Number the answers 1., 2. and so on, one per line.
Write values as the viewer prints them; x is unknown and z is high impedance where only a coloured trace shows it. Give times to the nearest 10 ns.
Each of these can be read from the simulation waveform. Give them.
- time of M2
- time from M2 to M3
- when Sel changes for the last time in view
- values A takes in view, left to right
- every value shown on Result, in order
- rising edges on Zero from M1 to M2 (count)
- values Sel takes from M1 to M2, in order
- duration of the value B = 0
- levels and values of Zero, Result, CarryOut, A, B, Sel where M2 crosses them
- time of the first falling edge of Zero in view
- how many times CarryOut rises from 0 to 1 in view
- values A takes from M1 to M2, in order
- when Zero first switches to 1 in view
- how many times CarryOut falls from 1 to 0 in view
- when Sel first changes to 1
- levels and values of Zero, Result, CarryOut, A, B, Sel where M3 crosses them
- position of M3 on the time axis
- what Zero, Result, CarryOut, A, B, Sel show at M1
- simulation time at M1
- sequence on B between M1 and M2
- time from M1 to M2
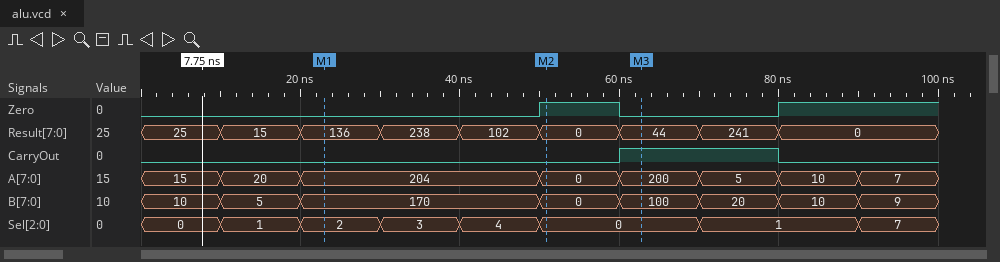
1. 50 ns
2. 10 ns
3. 90 ns
4. 15, 20, 204, 0, 200, 5, 10, 7
5. 25, 15, 136, 238, 102, 0, 44, 241, 0
6. 1
7. 2, 3, 4, 0
8. 10 ns
9. Zero=1, Result=0, CarryOut=0, A=0, B=0, Sel=0
10. 60 ns
11. 1
12. 204, 0
13. 50 ns
14. 1
15. 10 ns
16. Zero=0, Result=44, CarryOut=1, A=200, B=100, Sel=0
17. 60 ns
18. Zero=0, Result=136, CarryOut=0, A=204, B=170, Sel=2
19. 20 ns
20. 170, 0
21. 30 ns
